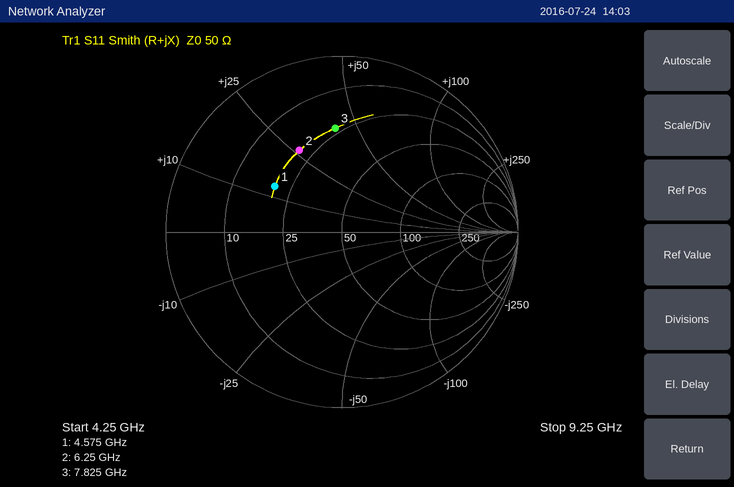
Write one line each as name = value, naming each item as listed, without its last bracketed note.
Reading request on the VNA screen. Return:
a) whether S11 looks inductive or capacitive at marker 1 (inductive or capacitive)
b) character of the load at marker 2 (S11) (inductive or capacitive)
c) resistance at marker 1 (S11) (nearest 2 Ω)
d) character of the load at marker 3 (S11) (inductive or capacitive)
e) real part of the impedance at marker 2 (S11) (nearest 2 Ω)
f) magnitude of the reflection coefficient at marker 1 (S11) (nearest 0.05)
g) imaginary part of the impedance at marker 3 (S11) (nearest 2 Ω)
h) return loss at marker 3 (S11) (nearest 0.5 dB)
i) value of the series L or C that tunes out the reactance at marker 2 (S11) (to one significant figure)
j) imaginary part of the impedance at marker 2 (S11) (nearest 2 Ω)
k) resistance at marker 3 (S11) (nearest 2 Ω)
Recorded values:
whether S11 looks inductive or capacitive at marker 1 = inductive
character of the load at marker 2 (S11) = inductive
resistance at marker 1 (S11) = 20 Ω
character of the load at marker 3 (S11) = inductive
real part of the impedance at marker 2 (S11) = 20 Ω
magnitude of the reflection coefficient at marker 1 (S11) = 0.45
imaginary part of the impedance at marker 3 (S11) = +42 Ω
return loss at marker 3 (S11) = 4.5 dB
value of the series L or C that tunes out the reactance at marker 2 (S11) = 1.0 pF
imaginary part of the impedance at marker 2 (S11) = +26 Ω
resistance at marker 3 (S11) = 22 Ω
